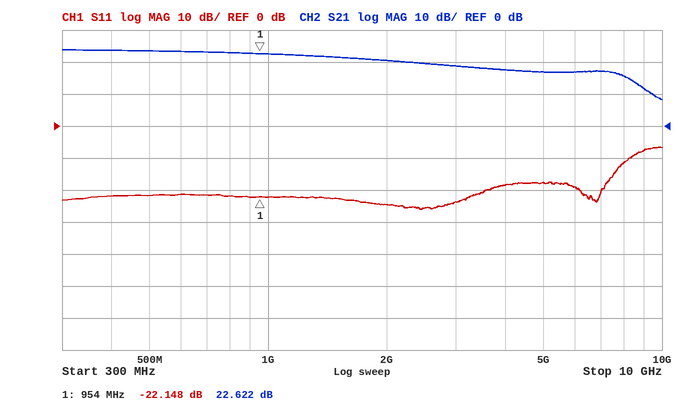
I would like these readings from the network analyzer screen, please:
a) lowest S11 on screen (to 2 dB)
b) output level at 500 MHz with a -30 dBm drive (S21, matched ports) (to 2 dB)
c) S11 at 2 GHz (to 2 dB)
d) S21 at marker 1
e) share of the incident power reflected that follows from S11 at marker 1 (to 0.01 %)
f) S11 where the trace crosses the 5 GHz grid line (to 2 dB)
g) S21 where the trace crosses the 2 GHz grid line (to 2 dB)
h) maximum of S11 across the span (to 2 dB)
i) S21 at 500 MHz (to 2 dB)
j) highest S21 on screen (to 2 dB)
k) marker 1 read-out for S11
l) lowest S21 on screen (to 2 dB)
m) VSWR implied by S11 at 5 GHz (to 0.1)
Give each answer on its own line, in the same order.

-26 dB
-6 dBm
-24 dB
22.622 dB
0.61 %
-18 dB
20 dB
-6 dB
24 dB
24 dB
-22.148 dB
8 dB
1.3
